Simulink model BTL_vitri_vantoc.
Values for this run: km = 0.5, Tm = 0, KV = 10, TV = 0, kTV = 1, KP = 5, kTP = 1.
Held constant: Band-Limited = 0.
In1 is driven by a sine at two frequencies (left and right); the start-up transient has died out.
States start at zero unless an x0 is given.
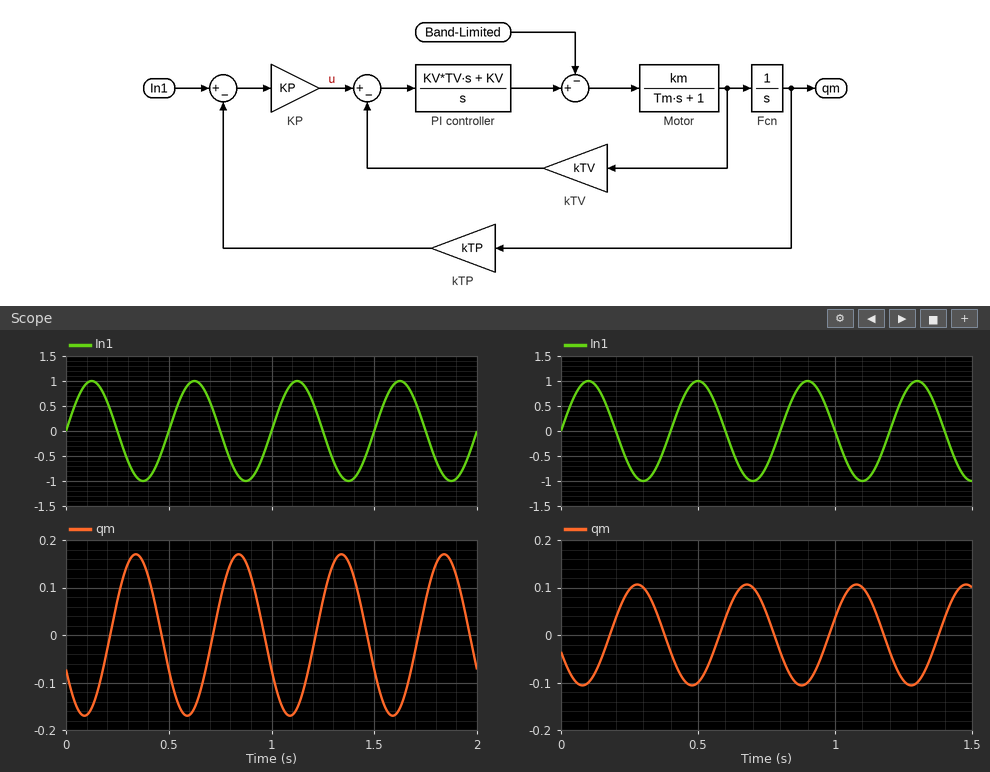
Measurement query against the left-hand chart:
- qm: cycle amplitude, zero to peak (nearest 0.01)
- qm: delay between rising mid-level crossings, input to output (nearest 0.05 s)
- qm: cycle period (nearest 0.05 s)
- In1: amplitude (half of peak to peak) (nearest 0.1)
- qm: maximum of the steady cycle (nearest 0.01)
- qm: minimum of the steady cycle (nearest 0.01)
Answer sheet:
0.17
0.20 s
0.50 s
1.0
0.17
-0.17
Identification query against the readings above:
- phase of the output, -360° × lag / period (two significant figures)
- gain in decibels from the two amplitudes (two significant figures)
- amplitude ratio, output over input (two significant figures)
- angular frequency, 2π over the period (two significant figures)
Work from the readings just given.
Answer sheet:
-140°
-15 dB
0.17
13 rad/s
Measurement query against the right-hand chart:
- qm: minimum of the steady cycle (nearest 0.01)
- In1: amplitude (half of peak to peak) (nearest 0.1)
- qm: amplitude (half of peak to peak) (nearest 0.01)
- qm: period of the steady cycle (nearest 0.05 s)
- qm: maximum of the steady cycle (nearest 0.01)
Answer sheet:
-0.11
1.0
0.11
0.40 s
0.11
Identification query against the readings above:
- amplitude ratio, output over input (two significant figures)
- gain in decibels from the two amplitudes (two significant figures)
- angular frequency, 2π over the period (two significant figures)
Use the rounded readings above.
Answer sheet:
0.11
-19 dB
16 rad/s
